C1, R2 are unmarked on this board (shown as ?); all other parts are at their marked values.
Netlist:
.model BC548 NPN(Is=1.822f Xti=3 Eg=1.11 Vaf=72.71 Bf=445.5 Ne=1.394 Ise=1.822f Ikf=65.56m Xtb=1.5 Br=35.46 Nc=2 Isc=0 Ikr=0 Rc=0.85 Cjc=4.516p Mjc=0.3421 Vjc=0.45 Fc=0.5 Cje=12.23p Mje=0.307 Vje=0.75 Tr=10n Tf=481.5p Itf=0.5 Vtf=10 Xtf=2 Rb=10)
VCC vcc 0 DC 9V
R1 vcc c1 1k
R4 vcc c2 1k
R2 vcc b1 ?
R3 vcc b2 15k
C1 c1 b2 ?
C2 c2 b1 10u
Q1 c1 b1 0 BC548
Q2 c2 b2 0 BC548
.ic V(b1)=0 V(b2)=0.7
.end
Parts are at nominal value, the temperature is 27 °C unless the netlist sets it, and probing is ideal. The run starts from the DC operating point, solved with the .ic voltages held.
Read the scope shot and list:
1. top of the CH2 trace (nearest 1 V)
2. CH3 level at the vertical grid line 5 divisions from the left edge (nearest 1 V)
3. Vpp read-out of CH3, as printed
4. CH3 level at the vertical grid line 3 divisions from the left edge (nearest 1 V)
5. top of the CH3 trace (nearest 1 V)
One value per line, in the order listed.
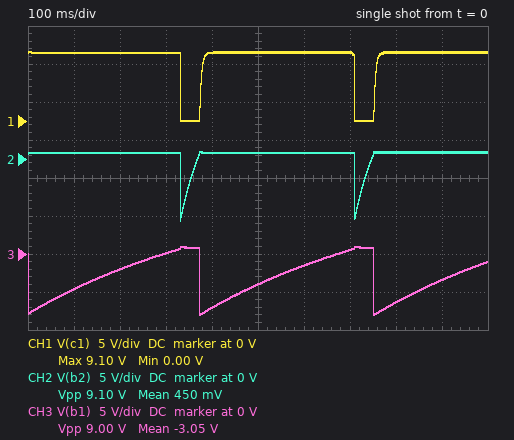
1 V
-4 V
9.00 V
0 V
1 V
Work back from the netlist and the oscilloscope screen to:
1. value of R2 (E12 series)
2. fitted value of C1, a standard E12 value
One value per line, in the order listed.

47 kΩ
3.9 µF
